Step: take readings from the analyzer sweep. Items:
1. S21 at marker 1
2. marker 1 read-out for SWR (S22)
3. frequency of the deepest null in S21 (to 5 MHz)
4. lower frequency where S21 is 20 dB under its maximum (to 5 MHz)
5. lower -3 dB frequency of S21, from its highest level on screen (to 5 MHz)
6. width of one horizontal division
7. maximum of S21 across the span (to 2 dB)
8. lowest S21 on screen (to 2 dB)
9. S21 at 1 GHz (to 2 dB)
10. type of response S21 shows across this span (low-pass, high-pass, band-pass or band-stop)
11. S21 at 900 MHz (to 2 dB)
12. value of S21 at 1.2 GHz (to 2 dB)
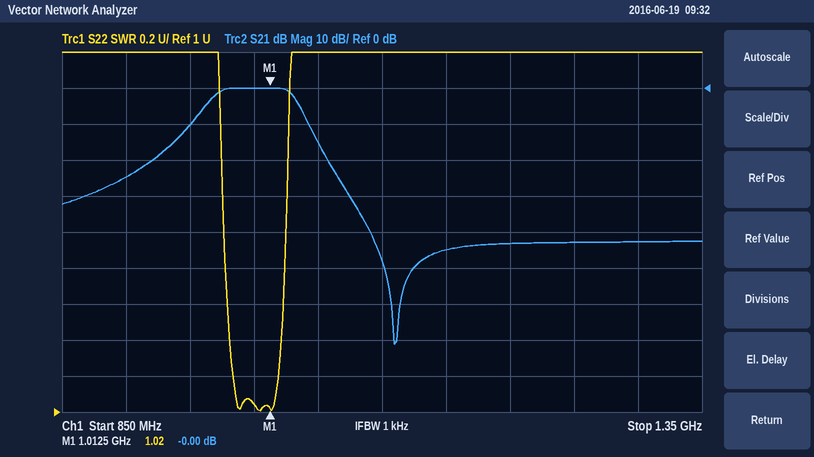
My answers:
-0.00 dB
1.02
1.110 GHz
920 MHz
965 MHz
50 MHz
0 dB
-72 dB
0 dB
band-pass
-24 dB
-44 dB
